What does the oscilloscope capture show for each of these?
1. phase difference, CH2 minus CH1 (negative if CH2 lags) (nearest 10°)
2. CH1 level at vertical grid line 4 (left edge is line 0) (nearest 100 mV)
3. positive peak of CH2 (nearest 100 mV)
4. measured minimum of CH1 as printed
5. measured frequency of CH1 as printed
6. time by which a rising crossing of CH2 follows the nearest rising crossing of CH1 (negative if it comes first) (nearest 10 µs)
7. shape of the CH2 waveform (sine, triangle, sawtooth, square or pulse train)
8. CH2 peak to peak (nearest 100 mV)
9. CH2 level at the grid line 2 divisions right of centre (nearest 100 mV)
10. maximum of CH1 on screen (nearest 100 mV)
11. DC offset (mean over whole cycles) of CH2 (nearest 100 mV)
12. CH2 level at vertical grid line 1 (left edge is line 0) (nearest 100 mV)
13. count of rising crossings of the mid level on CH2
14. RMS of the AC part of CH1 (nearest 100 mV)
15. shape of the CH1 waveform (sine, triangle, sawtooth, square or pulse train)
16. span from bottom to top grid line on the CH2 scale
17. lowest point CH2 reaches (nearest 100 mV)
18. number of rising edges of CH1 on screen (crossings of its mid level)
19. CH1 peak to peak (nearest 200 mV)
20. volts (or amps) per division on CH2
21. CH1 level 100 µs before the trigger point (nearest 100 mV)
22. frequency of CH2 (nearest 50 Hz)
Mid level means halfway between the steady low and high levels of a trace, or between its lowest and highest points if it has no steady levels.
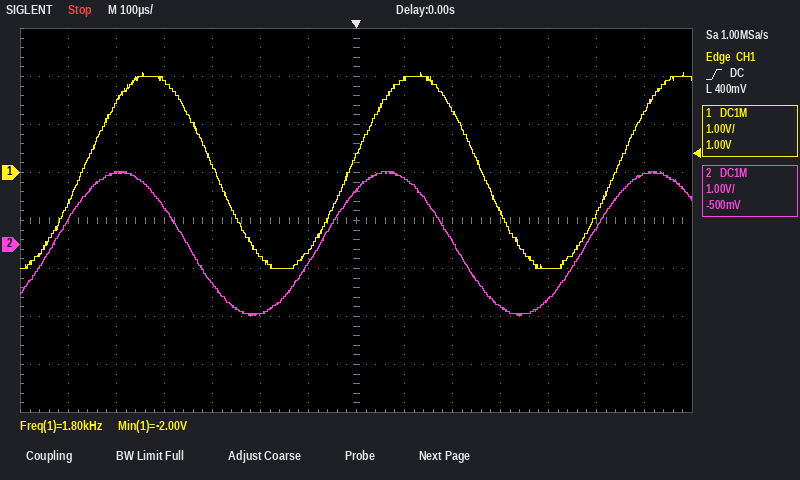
+40°
200 mV
1.5 V
-2.00 V
1.80 kHz
-60 µs
sine
3.0 V
100 mV
2.1 V
0.0 V
500 mV
3
1.4 V
sine
8 V
-1.5 V
3
4.0 V
1 V
-1.6 V
1.80 kHz
